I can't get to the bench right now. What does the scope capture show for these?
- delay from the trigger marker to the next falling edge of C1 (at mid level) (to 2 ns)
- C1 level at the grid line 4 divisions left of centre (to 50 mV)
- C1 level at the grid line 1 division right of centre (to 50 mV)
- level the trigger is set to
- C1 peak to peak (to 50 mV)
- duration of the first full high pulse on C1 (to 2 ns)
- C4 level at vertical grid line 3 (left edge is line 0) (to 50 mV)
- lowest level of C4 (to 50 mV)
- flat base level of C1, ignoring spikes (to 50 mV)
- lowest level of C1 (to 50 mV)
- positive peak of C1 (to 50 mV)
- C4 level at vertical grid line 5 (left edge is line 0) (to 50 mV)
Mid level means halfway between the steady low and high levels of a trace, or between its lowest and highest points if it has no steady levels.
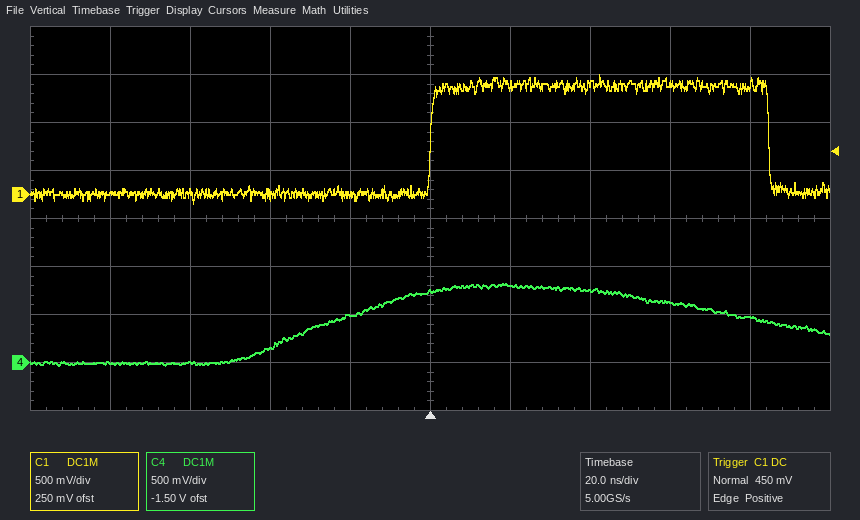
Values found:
84 ns
0 mV
1.15 V
450 mV
1.35 V
84 ns
150 mV
-50 mV
0 mV
-100 mV
1.25 V
750 mV
